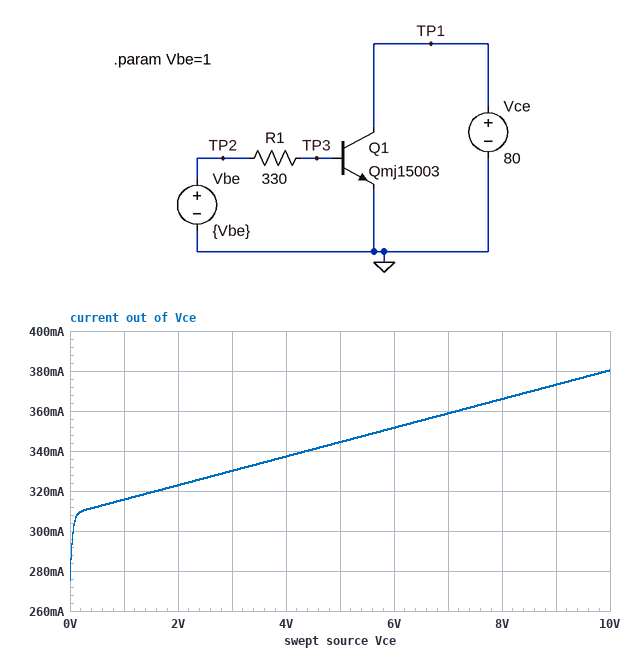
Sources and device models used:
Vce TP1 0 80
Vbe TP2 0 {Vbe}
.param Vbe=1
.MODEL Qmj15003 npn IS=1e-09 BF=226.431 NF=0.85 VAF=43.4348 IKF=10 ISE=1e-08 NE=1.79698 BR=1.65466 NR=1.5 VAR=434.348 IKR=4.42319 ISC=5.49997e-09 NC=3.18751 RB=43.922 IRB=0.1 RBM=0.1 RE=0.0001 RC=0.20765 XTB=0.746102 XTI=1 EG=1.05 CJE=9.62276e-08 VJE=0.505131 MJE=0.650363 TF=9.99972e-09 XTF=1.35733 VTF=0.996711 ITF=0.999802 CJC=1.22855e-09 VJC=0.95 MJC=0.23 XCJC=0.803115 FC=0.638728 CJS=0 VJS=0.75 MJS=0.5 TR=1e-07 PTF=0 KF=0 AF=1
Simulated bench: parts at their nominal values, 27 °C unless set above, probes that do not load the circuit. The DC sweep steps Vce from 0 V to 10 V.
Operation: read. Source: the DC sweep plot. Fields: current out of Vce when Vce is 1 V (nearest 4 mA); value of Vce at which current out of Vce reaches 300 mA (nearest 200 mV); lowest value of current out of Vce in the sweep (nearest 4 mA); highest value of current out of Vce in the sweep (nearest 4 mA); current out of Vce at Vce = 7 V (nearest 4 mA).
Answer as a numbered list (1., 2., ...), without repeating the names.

1. 316 mA
2. 0 V
3. 276 mA
4. 380 mA
5. 360 mA
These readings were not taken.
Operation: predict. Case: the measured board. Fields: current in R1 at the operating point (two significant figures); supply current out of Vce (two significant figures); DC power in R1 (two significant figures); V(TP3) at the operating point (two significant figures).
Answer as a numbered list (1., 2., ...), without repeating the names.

1. 1.5 mA
2. 880 mA
3. 770 µW
4. 500 mV
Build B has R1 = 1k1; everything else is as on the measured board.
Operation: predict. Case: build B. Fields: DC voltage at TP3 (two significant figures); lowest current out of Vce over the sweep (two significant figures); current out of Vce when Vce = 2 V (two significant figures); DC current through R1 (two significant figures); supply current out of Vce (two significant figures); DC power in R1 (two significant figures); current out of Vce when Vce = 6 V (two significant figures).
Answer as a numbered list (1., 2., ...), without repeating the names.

1. 430 mV
2. 95 mA
3. 110 mA
4. 520 µA
5. 290 mA
6. 300 µW
7. 120 mA
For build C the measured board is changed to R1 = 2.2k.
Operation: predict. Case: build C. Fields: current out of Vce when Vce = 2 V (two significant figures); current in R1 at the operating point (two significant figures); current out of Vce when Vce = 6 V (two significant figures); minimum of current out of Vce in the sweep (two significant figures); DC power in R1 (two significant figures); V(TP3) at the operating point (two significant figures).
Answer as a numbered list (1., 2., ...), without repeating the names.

1. 53 mA
2. 270 µA
3. 58 mA
4. 47 mA
5. 160 µW
6. 400 mV
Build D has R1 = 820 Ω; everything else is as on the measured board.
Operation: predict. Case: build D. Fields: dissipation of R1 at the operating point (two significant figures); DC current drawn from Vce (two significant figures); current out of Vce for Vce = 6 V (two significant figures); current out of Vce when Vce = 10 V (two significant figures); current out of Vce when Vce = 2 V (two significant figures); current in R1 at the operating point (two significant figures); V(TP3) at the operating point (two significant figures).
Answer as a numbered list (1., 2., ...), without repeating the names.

1. 380 µW
2. 390 mA
3. 150 mA
4. 170 mA
5. 140 mA
6. 680 µA
7. 440 mV
